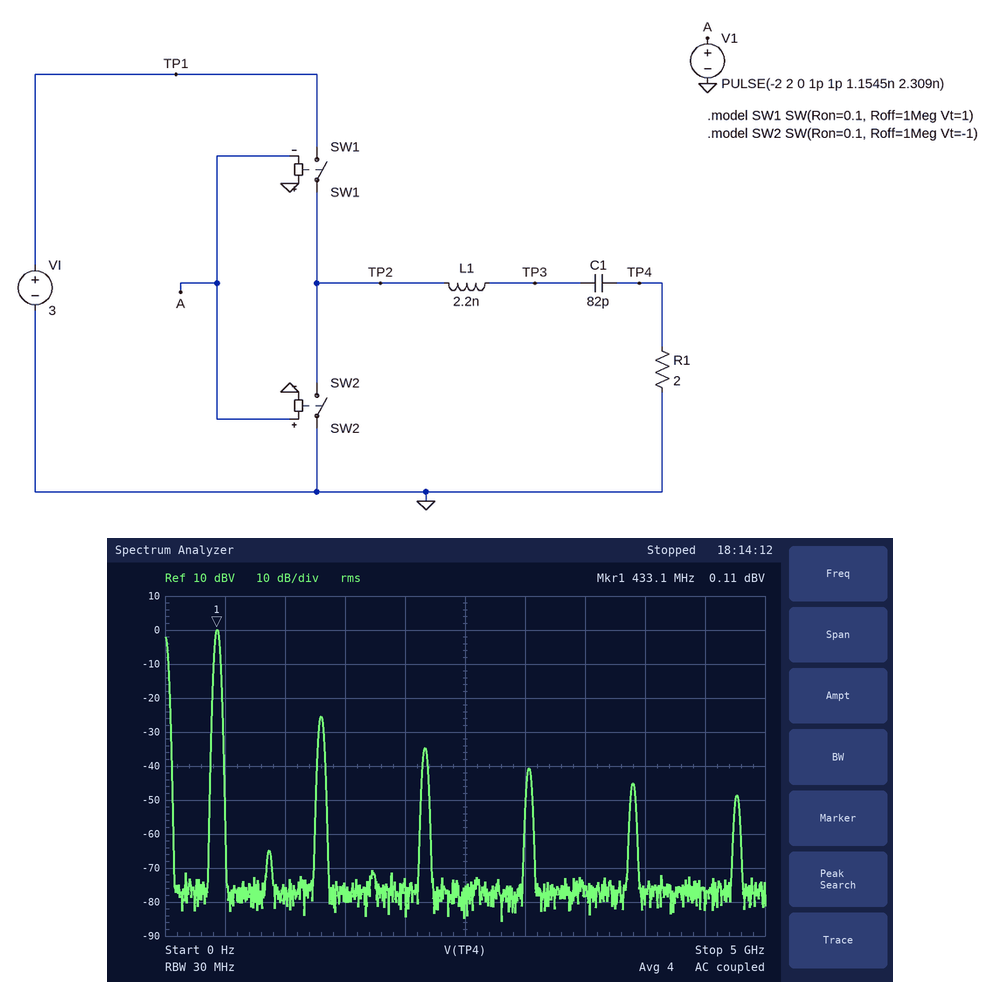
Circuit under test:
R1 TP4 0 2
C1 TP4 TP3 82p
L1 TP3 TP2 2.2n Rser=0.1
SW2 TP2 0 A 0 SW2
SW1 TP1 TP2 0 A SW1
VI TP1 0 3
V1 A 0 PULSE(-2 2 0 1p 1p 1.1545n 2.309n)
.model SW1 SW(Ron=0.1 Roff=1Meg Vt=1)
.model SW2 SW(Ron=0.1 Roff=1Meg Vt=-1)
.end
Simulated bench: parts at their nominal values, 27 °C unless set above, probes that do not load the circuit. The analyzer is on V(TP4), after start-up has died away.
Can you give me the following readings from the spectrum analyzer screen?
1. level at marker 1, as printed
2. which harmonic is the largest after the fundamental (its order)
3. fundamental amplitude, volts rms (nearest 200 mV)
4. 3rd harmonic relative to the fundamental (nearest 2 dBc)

0.11 dBV
3
1.0 V
-26 dBc
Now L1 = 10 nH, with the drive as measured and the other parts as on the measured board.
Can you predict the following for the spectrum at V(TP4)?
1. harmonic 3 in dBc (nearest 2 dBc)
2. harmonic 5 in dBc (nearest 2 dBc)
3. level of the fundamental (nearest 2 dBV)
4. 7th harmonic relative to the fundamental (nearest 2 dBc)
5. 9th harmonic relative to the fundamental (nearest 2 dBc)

-20 dBc
-30 dBc
-18 dBV
-36 dBc
-40 dBc
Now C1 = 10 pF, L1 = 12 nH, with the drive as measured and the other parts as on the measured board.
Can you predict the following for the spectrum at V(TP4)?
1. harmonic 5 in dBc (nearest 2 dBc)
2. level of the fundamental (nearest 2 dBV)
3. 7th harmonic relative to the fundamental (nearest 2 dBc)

-44 dBc
-4 dBV
-50 dBc
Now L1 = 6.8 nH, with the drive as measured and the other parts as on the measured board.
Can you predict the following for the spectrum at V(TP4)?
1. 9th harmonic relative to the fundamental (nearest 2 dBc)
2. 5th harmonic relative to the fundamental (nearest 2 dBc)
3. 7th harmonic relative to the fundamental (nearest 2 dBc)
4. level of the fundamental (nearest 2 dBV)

-40 dBc
-30 dBc
-36 dBc
-14 dBV
